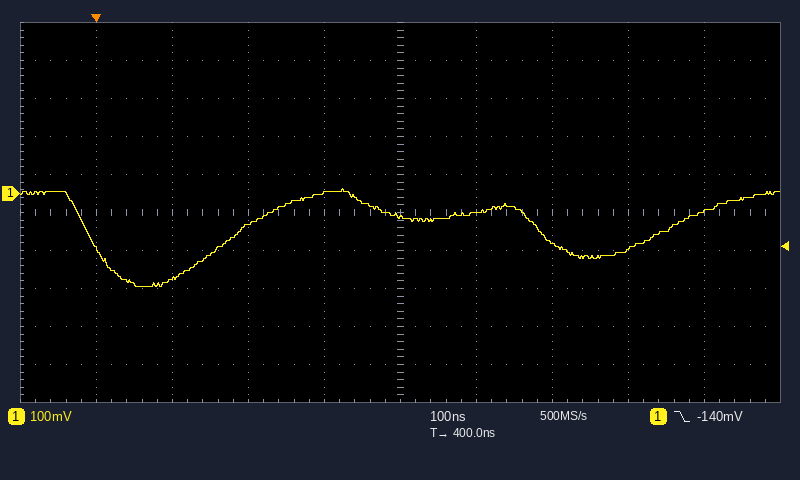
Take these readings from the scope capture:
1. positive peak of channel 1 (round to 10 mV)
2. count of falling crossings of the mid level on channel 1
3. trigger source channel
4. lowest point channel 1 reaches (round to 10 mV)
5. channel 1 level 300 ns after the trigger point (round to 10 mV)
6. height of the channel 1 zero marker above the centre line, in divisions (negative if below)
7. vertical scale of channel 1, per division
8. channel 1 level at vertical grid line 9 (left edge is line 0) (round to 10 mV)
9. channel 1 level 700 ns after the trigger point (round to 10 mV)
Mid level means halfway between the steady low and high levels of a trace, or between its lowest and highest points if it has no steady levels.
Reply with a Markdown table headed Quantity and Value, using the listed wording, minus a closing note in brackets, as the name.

| Quantity | Value |
|---|---|
| positive peak of channel 1 | 10 mV |
| count of falling crossings of the mid level on channel 1 | 2 |
| trigger source channel | channel 1 |
| lowest point channel 1 reaches | -240 mV |
| channel 1 level 300 ns after the trigger point | 0 mV |
| height of the channel 1 zero marker above the centre line, in divisions | +0.5 div |
| vertical scale of channel 1, per division | 100 mV |
| channel 1 level at vertical grid line 9 (left edge is line 0) | -50 mV |
| channel 1 level 700 ns after the trigger point | -150 mV |
